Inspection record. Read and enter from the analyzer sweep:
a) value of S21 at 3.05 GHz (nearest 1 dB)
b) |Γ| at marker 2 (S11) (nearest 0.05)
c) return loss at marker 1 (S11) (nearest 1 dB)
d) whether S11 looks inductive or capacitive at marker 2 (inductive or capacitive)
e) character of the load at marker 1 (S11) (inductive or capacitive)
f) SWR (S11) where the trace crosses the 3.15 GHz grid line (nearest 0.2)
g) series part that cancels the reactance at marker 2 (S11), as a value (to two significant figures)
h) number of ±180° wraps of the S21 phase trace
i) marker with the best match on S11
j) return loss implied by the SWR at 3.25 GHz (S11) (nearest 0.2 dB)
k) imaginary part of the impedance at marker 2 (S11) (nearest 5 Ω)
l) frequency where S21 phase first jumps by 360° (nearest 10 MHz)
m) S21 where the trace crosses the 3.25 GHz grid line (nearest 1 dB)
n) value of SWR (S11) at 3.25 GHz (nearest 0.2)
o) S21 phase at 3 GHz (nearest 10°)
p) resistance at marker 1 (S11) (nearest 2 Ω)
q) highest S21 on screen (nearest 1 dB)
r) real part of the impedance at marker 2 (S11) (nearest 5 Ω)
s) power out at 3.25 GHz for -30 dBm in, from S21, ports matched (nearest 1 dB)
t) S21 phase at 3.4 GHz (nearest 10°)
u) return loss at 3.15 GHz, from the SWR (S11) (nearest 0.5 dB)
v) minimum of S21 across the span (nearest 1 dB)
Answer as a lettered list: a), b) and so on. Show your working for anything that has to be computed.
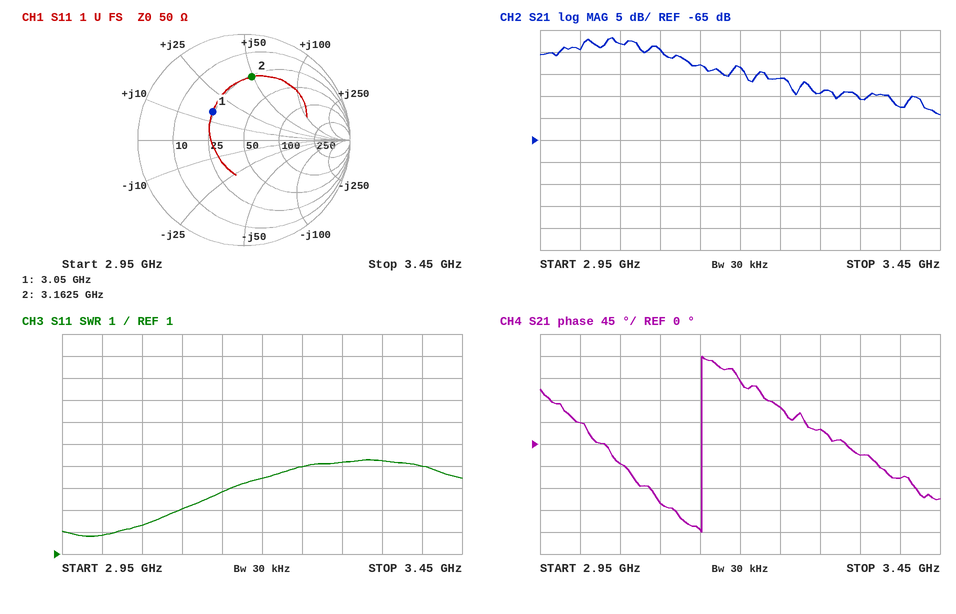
a) -43 dB
b) 0.60
c) 8 dB
d) inductive
e) inductive
f) 3.8
g) C = 1/(2π × 3.1625 GHz × 50 Ω) ≈ 1.0 pF
h) 1
i) marker 1
j) −20 log10((5 − 1)/(5 + 1)) ≈ 3.52 dB, so 3.6 dB to the nearest 0.2 dB
k) +50 Ω
l) 3.15 GHz
m) -51 dB
n) 5.0
o) 40°
p) 24 Ω
q) -42 dB
r) 25 Ω
s) -30 dBm + (-51 dB) = -81 dBm
t) -70°
u) −20 log10((3.8 − 1)/(3.8 + 1)) ≈ 4.68 dB, so 4.5 dB to the nearest 0.5 dB
v) -59 dB
